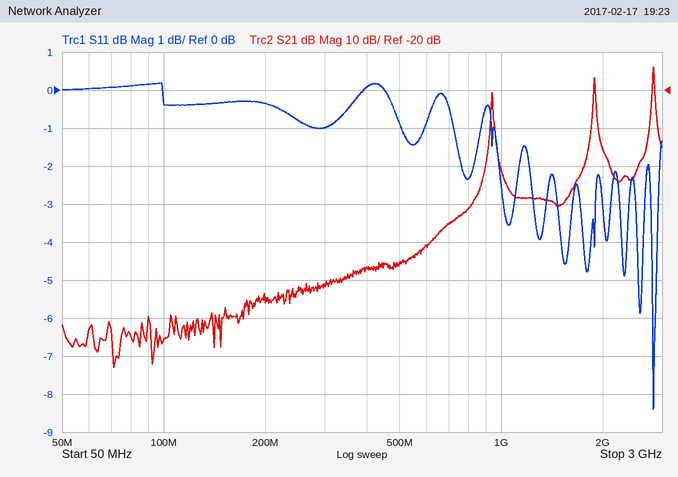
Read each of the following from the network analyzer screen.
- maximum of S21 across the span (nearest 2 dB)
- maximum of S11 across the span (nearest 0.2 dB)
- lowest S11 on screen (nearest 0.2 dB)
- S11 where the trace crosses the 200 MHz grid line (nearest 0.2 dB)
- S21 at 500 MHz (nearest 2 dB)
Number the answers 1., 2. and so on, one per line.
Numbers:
1. -14 dB
2. 0.2 dB
3. -8.4 dB
4. -0.4 dB
5. -66 dB
